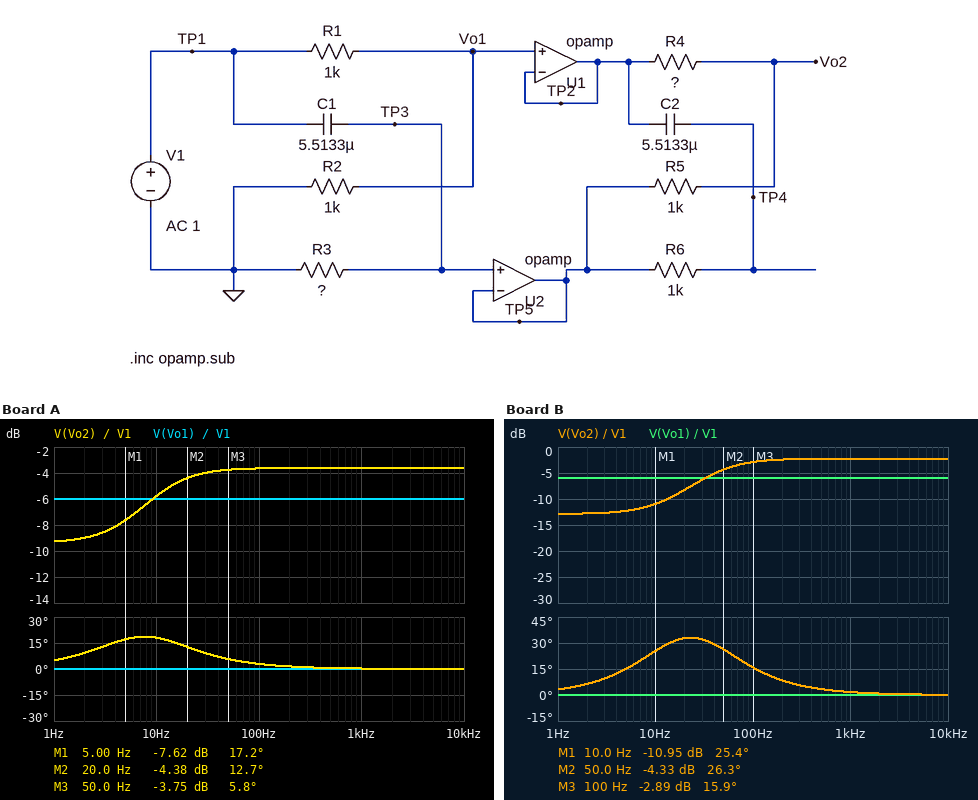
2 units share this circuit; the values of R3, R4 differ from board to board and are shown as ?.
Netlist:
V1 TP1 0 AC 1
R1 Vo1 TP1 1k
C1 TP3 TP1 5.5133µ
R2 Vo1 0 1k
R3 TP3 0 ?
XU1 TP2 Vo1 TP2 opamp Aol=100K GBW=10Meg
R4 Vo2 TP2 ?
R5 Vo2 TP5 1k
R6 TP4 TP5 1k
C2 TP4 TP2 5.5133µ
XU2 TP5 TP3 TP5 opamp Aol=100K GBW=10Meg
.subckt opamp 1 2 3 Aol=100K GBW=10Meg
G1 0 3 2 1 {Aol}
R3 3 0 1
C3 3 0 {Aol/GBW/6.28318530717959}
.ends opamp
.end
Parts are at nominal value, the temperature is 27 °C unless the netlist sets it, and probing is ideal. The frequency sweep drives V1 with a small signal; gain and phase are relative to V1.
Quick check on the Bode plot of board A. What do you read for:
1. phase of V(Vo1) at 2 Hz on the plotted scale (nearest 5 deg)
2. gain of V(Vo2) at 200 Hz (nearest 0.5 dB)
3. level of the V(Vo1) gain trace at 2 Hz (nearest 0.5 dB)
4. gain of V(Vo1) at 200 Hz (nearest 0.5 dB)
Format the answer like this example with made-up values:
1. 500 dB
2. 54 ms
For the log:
1. 0 deg
2. -3.5 dB
3. -6.0 dB
4. -6.0 dB
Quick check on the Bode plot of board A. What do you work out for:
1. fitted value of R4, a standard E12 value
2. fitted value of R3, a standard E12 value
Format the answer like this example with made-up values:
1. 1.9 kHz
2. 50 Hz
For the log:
1. 470 Ω
2. 2.7 kΩ
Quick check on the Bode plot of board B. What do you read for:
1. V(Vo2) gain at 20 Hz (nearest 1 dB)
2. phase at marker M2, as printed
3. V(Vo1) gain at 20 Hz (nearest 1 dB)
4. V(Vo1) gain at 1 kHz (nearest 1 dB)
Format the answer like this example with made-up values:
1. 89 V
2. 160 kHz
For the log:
1. -8 dB
2. 26.3 deg
3. -6 dB
4. -6 dB
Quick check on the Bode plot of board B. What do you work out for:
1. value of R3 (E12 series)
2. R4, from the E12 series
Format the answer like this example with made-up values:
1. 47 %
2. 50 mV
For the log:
1. 680 Ω
2. 1.2 kΩ
